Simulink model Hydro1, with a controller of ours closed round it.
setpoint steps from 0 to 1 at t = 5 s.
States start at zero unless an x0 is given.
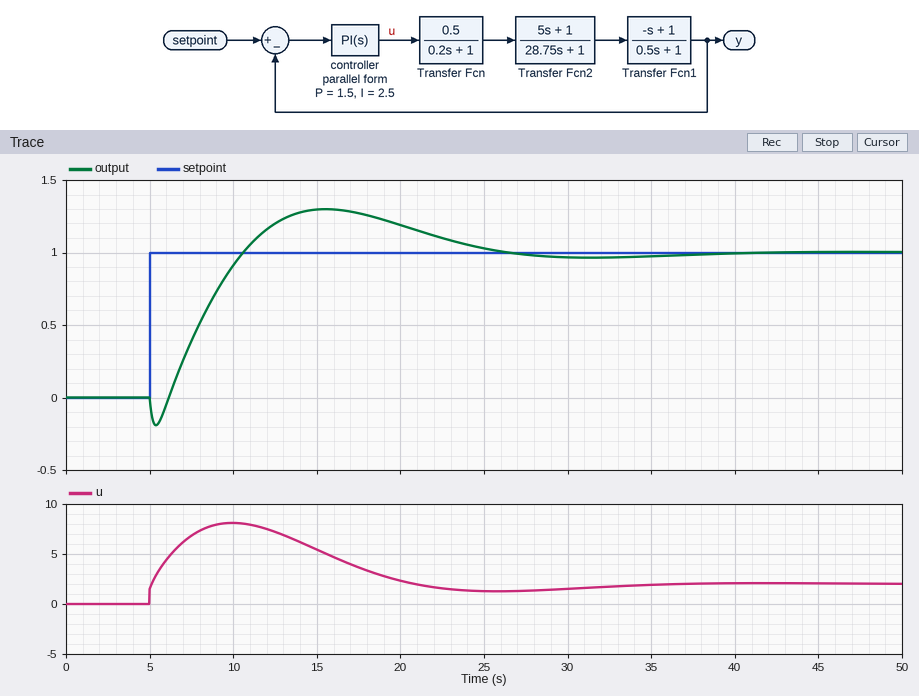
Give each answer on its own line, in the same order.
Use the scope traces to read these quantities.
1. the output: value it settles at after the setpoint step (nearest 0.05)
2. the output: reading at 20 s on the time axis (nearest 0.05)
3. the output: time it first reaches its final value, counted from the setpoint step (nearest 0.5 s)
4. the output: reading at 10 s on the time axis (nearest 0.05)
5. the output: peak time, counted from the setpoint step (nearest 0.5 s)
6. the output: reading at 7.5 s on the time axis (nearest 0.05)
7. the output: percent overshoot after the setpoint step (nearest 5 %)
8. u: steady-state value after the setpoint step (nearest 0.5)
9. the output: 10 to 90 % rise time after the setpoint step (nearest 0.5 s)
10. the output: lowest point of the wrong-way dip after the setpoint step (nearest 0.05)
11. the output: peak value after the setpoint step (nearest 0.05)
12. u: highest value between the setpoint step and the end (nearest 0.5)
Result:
1.00
1.20
5.5 s
0.90
10.5 s
0.40
30 %
2.0
3.5 s
-0.20
1.30
8.0
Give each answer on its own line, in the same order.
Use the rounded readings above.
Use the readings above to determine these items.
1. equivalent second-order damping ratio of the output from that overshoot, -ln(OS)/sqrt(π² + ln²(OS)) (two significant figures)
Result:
0.36
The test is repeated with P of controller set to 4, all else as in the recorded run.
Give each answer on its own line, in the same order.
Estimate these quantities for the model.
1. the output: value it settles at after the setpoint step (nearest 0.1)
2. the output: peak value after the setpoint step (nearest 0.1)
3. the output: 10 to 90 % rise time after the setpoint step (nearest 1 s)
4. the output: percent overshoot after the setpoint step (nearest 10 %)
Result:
1.0
1.2
4 s
20 %
